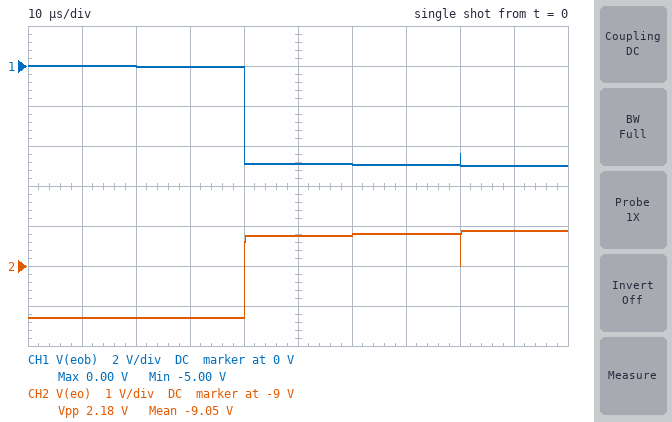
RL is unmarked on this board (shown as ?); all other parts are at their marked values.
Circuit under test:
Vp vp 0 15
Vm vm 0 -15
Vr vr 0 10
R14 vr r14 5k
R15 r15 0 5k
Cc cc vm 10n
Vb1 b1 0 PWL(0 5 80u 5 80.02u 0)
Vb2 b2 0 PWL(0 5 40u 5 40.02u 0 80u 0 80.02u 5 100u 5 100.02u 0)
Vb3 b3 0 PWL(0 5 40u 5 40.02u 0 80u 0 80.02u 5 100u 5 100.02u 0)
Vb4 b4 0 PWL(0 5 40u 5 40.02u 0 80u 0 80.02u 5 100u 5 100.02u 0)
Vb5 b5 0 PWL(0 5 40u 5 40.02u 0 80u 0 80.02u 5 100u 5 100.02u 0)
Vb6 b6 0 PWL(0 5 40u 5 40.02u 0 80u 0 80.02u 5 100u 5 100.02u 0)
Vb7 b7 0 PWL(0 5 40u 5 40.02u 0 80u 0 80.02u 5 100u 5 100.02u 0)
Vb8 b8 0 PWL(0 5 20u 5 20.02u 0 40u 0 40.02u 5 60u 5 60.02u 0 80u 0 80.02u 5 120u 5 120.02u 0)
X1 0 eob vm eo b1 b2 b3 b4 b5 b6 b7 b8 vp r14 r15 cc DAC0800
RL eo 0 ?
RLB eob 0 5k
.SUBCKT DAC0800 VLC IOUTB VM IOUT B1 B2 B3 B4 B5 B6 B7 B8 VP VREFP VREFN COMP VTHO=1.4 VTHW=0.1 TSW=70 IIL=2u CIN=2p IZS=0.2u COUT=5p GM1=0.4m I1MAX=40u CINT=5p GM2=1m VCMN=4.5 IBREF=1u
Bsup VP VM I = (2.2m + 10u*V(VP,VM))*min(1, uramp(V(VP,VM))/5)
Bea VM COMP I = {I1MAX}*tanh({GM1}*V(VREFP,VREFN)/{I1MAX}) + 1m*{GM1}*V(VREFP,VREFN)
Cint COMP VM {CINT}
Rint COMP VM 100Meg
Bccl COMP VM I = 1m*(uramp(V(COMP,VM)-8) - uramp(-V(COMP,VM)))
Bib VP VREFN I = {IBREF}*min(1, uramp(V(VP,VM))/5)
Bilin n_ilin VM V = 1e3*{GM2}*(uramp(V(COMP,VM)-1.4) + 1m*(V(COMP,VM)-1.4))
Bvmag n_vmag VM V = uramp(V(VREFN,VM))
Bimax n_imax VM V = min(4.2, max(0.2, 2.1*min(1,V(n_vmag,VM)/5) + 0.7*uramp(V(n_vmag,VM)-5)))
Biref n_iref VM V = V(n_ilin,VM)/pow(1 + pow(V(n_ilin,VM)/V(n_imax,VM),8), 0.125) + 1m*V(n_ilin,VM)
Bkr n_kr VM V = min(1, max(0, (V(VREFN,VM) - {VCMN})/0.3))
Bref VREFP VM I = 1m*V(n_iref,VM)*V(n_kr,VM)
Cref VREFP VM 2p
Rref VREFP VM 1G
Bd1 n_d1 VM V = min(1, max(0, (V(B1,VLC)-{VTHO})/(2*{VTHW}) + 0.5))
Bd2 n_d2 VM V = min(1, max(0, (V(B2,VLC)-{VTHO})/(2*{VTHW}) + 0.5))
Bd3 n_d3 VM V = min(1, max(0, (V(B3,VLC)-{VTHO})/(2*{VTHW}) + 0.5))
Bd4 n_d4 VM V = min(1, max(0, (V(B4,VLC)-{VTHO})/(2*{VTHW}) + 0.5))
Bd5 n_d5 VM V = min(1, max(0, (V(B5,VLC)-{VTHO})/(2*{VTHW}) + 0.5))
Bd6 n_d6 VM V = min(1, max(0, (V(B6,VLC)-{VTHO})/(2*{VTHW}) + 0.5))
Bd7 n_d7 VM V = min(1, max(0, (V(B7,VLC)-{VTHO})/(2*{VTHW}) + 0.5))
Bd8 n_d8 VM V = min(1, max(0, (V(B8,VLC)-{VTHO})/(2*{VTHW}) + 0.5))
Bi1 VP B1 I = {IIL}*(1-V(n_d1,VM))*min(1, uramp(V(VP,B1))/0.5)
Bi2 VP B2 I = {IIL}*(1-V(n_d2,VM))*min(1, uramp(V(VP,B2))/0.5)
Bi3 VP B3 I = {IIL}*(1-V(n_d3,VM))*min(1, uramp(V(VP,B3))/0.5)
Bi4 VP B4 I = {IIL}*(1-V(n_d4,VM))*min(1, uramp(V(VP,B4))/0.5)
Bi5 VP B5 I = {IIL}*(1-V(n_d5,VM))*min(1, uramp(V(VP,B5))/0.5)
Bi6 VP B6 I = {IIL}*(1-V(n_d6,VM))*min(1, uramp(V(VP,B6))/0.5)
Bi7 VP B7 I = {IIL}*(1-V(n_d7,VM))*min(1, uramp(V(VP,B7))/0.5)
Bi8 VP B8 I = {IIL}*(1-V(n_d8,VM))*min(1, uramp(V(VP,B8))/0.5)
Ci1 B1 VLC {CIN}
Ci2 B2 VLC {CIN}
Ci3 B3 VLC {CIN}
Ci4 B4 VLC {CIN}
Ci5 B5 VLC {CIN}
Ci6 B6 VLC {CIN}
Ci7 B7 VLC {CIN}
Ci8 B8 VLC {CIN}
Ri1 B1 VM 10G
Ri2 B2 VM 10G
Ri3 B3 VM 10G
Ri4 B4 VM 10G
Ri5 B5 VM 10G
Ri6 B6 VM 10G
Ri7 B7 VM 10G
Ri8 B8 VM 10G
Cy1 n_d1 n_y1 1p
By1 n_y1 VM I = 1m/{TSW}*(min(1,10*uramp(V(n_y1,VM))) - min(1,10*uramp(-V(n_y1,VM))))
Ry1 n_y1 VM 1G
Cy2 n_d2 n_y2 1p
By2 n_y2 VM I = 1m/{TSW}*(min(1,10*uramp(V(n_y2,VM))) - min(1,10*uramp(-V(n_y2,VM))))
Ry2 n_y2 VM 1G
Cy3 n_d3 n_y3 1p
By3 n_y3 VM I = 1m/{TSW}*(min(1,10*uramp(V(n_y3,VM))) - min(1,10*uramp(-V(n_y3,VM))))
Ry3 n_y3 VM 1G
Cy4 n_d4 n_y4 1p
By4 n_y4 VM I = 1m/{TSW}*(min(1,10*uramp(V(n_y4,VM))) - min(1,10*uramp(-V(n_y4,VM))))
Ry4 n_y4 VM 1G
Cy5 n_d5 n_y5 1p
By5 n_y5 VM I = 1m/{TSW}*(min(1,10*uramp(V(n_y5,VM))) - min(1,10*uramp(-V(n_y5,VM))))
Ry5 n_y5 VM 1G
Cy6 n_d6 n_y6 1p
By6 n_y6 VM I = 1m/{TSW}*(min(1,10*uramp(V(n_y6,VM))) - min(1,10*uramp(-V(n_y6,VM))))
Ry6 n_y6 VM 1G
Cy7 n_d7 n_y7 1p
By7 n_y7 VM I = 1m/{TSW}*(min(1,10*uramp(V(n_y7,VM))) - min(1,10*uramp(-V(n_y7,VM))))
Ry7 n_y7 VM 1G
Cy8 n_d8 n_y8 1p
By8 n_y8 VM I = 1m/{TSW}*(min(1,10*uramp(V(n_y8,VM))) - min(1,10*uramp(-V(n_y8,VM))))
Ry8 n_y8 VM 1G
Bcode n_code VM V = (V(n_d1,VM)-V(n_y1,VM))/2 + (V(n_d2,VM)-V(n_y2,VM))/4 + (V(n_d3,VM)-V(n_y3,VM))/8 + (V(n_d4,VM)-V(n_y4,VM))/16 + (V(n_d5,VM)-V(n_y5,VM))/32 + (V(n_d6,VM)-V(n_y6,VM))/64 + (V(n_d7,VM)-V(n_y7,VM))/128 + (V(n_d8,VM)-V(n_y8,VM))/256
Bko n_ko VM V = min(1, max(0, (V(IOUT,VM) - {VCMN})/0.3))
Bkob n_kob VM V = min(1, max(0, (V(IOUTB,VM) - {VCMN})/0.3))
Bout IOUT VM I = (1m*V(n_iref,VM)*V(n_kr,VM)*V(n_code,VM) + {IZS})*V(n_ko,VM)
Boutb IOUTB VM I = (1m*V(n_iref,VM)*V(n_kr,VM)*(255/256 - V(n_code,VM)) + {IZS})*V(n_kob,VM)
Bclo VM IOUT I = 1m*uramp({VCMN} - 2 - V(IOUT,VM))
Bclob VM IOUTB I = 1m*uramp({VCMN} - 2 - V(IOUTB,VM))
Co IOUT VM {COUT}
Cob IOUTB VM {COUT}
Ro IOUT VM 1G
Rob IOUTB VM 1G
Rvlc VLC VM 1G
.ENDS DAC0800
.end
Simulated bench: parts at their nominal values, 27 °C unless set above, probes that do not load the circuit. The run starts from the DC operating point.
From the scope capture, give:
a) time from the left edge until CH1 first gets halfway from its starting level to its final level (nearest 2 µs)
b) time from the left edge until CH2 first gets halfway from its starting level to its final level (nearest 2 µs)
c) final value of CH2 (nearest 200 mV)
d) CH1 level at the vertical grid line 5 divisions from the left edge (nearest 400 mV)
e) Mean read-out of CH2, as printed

40 µs
40 µs
-8.2 V
-4.8 V
-9.05 V
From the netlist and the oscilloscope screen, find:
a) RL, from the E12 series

8.2 kΩ
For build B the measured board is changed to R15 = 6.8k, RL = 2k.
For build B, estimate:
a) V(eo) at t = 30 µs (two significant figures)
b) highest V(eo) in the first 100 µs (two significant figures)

-4.0 V
-2.0 V
